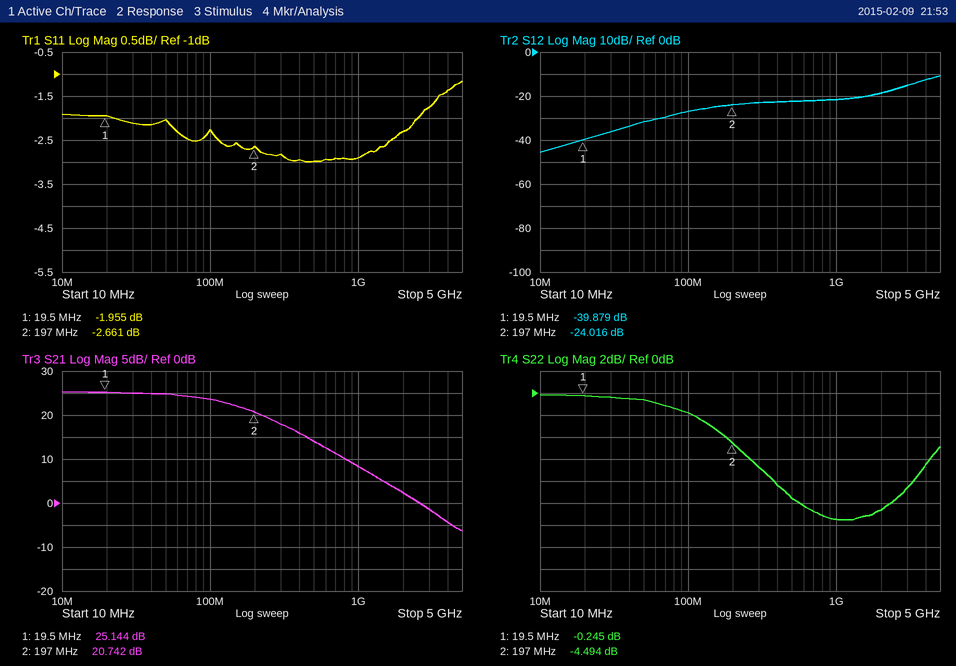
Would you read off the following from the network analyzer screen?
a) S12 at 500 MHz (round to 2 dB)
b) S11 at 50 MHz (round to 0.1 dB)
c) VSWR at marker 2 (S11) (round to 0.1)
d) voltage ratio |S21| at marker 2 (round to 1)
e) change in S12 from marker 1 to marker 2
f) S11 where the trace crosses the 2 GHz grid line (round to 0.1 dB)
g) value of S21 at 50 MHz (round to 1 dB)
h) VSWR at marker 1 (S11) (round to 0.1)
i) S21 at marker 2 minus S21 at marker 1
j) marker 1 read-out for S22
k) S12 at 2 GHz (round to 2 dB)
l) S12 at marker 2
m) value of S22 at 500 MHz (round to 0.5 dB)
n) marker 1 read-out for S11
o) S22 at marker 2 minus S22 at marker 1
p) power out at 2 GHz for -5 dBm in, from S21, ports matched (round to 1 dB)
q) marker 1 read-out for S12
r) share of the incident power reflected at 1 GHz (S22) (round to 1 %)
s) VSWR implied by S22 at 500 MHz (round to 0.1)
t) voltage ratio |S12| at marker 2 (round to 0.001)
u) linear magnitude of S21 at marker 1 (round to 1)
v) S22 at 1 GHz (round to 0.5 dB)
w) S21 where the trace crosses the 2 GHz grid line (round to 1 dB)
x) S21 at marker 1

-22 dB
-2.0 dB
6.6
11
15.863 dB
-2.3 dB
25 dB
8.9
-4.402 dB
-0.245 dB
-18 dB
-24.016 dB
-9.5 dB
-1.955 dB
-4.249 dB
-3 dBm
-39.879 dB
7 %
2.0
0.063
18
-11.5 dB
2 dB
25.144 dB
